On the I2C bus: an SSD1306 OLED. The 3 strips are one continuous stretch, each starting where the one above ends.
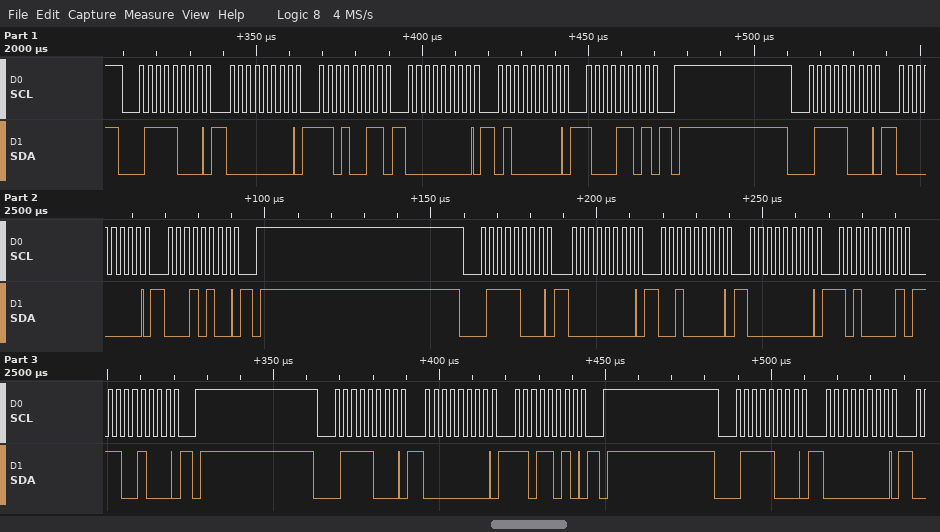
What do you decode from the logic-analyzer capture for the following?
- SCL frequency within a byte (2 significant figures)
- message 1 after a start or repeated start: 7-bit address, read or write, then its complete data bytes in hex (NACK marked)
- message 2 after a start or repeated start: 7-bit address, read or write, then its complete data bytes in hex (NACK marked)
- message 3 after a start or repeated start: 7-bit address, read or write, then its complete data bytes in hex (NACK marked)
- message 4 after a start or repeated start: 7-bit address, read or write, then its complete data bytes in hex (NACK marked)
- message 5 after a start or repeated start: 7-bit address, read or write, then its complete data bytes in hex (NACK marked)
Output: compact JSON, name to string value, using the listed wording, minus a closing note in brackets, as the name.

{"SCL frequency within a byte": "400 kHz", "message 1 after a start or repeated start: 7-bit address, read or write, then its complete data bytes in hex": "0x3C write: 00 D3 00 40 8D", "message 2 after a start or repeated start: 7-bit address, read or write, then its complete data bytes in hex": "0x3C write: 00 14", "message 3 after a start or repeated start: 7-bit address, read or write, then its complete data bytes in hex": "0x3C write: 00 20 00 A1 C8", "message 4 after a start or repeated start: 7-bit address, read or write, then its complete data bytes in hex": "0x3C write: 00 DA", "message 5 after a start or repeated start: 7-bit address, read or write, then its complete data bytes in hex": "0x3C write: 00"}
